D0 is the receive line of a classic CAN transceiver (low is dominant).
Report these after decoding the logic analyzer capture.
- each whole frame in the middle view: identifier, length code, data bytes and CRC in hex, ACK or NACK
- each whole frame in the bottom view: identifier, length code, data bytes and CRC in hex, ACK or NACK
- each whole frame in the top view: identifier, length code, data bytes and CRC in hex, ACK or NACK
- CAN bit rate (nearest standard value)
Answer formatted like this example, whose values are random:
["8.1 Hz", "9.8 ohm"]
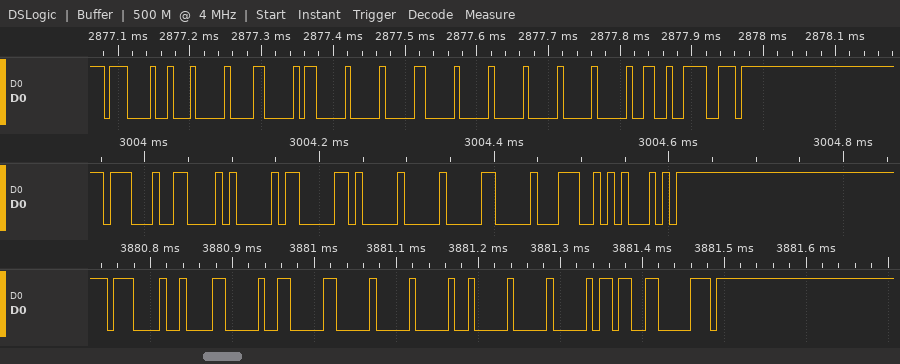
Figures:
["ID 713, DLC 5, data 03 05 00 01 00, CRC 72A2, ACK", "ID 709, DLC 6, data 03 04 00 01 00 00, CRC 6CC1, ACK", "ID 709, DLC 8, data 03 03 00 01 00 00 00 00, CRC 64F3, ACK", "125 kbit/s"]
